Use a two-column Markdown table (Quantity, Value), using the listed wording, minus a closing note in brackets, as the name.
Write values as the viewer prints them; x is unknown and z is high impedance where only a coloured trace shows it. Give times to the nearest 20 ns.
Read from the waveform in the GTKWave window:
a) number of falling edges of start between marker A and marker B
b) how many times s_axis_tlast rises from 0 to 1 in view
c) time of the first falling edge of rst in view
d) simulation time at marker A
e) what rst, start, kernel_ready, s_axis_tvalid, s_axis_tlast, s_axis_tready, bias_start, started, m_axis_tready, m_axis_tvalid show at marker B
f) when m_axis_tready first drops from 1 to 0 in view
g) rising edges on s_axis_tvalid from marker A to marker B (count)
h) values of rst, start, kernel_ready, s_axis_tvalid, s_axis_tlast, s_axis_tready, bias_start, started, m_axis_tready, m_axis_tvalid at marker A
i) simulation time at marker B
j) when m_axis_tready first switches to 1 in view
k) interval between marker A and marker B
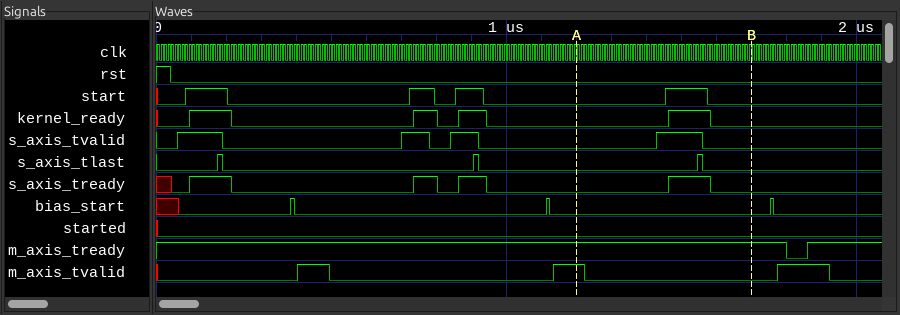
| Quantity | Value |
|---|---|
| number of falling edges of start between marker A and marker B | 1 |
| how many times s_axis_tlast rises from 0 to 1 in view | 3 |
| time of the first falling edge of rst in view | 40 ns |
| simulation time at marker A | 1200 ns |
| what rst, start, kernel_ready, s_axis_tvalid, s_axis_tlast, s_axis_tready, bias_start, started, m_axis_tready, m_axis_tvalid show at marker B | rst=0, start=0, kernel_ready=0, s_axis_tvalid=0, s_axis_tlast=0, s_axis_tready=0, bias_start=0, started=0, m_axis_tready=1, m_axis_tvalid=0 |
| when m_axis_tready first drops from 1 to 0 in view | 1800 ns |
| rising edges on s_axis_tvalid from marker A to marker B | 1 |
| values of rst, start, kernel_ready, s_axis_tvalid, s_axis_tlast, s_axis_tready, bias_start, started, m_axis_tready, m_axis_tvalid at marker A | rst=0, start=0, kernel_ready=0, s_axis_tvalid=0, s_axis_tlast=0, s_axis_tready=0, bias_start=0, started=0, m_axis_tready=1, m_axis_tvalid=1 |
| simulation time at marker B | 1700 ns |
| when m_axis_tready first switches to 1 in view | 1860 ns |
| interval between marker A and marker B | 500 ns |
